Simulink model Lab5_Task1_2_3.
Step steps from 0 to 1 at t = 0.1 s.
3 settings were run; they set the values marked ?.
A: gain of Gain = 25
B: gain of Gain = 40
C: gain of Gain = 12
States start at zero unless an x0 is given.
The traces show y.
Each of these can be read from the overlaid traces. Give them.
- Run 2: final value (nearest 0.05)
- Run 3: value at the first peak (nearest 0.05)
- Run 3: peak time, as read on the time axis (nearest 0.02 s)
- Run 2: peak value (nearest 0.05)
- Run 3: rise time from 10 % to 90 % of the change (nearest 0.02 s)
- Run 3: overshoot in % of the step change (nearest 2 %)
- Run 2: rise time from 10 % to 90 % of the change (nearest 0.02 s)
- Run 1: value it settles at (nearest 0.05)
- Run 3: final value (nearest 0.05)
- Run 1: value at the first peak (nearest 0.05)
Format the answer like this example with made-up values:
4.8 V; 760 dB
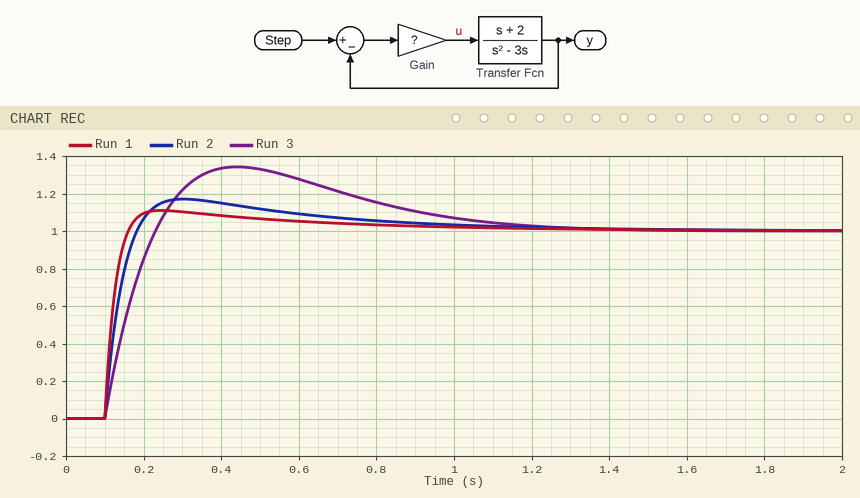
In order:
1.00; 1.35; 0.44 s; 1.15; 0.10 s; 34 %; 0.06 s; 1.00; 1.00; 1.10
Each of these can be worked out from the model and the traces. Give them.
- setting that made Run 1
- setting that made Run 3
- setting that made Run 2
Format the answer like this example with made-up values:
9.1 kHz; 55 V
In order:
B; C; A
